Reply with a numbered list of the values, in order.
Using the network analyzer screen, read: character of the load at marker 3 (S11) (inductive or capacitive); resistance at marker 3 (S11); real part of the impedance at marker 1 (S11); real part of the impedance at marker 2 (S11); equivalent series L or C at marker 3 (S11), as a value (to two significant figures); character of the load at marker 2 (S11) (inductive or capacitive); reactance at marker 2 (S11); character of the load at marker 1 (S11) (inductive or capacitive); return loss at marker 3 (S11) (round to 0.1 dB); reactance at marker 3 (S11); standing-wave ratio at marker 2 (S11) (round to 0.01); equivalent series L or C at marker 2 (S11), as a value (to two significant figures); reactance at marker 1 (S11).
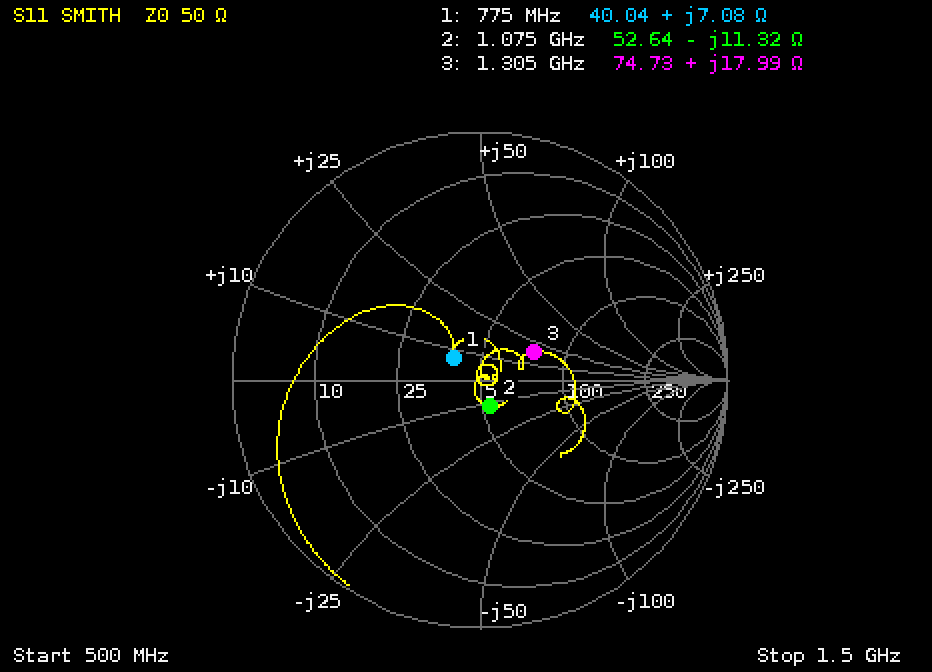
1. inductive
2. 74.73 Ω
3. 40.04 Ω
4. 52.64 Ω
5. 2.2 nH
6. capacitive
7. -11.32 Ω
8. inductive
9. 12.3 dB
10. +17.99 Ω
11. 1.25
12. 13 pF
13. +7.08 Ω
